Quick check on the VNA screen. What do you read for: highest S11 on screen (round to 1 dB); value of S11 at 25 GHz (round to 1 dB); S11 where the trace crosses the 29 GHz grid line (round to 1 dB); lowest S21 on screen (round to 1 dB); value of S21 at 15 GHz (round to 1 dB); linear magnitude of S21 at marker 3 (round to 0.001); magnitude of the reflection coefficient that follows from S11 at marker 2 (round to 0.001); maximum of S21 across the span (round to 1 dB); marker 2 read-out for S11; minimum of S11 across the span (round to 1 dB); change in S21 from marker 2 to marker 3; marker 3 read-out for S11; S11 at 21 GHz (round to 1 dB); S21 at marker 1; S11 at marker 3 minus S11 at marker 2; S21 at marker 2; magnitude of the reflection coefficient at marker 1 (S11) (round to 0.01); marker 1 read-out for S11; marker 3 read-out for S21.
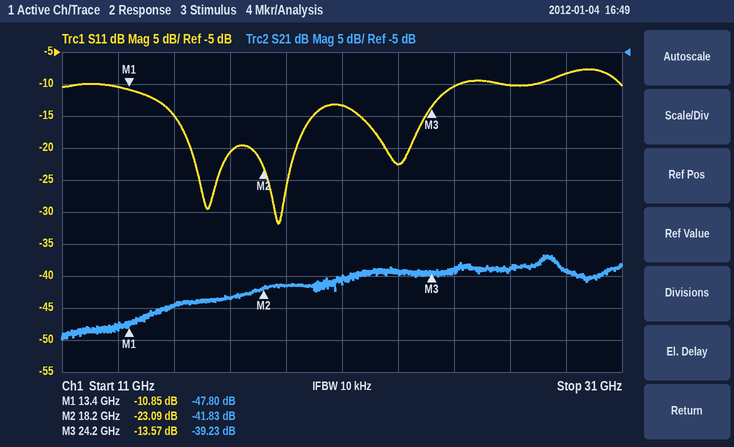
-8 dB
-10 dB
-8 dB
-50 dB
-45 dB
0.011
0.070
-37 dB
-23.09 dB
-32 dB
2.60 dB
-13.57 dB
-13 dB
-47.80 dB
9.52 dB
-41.83 dB
0.29
-10.85 dB
-39.23 dB
